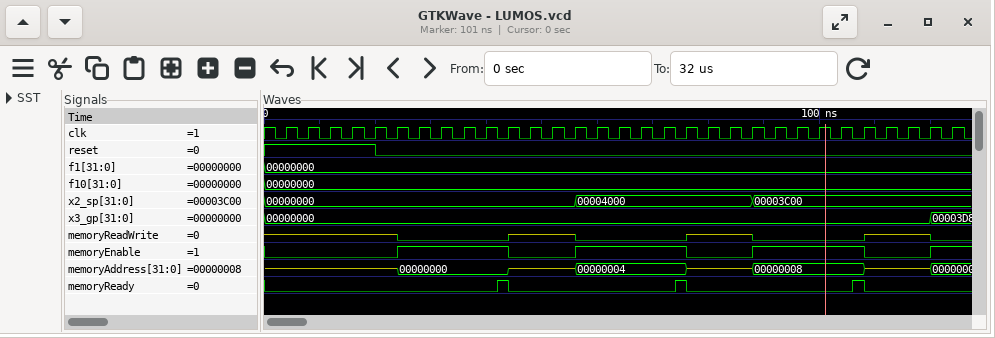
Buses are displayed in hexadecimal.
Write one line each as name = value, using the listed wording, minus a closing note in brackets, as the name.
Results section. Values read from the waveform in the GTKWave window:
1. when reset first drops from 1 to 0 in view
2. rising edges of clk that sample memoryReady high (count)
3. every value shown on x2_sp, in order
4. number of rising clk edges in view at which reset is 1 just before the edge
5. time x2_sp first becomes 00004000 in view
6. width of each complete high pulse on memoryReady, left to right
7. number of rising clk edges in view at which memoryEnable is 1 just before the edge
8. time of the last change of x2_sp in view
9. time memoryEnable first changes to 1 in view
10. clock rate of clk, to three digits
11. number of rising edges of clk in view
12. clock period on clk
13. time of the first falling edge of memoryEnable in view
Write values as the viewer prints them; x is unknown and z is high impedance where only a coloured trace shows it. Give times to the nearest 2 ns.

when reset first drops from 1 to 0 in view = 20 ns
rising edges of clk that sample memoryReady high = 3
every value shown on x2_sp, in order = 00000000, 00004000, 00003C00
number of rising clk edges in view at which reset is 1 just before the edge = 5
time x2_sp first becomes 00004000 in view = 56 ns
width of each complete high pulse on memoryReady, left to right = 2 ns, 2 ns, 2 ns
number of rising clk edges in view at which memoryEnable is 1 just before the edge = 16
time of the last change of x2_sp in view = 88 ns
time memoryEnable first changes to 1 in view = 24 ns
clock rate of clk, to three digits = 250 MHz
number of rising edges of clk in view = 31
clock period on clk = 4 ns
time of the first falling edge of memoryEnable in view = 44 ns
